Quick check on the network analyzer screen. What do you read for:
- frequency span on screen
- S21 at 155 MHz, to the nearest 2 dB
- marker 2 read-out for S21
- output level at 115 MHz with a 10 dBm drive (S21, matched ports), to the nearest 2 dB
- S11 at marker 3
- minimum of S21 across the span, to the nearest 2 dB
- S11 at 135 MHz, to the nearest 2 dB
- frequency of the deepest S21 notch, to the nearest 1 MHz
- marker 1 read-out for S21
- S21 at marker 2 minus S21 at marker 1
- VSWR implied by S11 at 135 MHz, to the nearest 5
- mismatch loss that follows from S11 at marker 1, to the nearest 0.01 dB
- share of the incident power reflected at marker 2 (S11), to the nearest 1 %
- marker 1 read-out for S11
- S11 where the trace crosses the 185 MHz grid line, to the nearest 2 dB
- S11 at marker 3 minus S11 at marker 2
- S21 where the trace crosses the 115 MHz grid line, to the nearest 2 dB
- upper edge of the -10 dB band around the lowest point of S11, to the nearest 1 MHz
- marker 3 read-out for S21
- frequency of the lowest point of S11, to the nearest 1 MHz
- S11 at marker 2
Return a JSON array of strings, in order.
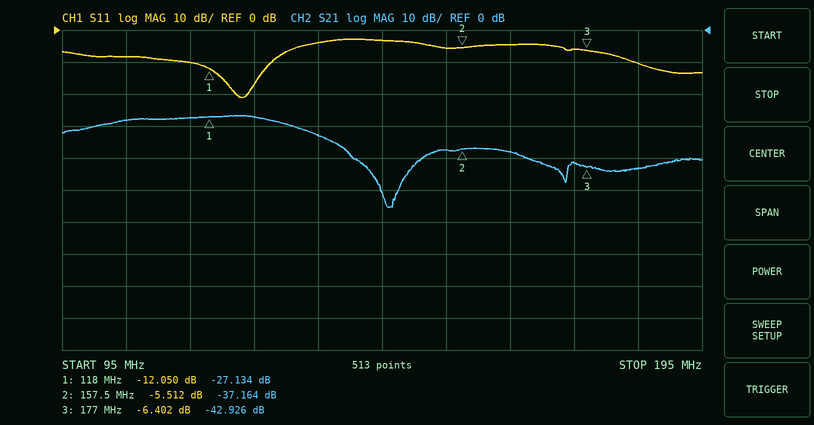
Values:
["100 MHz", "-38 dB", "-37.164 dB", "-18 dBm", "-6.402 dB", "-56 dB", "-4 dB", "146 MHz", "-27.134 dB", "-10.030 dB", "5", "0.28 dB", "28 %", "-12.050 dB", "-10 dB", "-0.890 dB", "-28 dB", "128 MHz", "-42.926 dB", "123 MHz", "-5.512 dB"]
